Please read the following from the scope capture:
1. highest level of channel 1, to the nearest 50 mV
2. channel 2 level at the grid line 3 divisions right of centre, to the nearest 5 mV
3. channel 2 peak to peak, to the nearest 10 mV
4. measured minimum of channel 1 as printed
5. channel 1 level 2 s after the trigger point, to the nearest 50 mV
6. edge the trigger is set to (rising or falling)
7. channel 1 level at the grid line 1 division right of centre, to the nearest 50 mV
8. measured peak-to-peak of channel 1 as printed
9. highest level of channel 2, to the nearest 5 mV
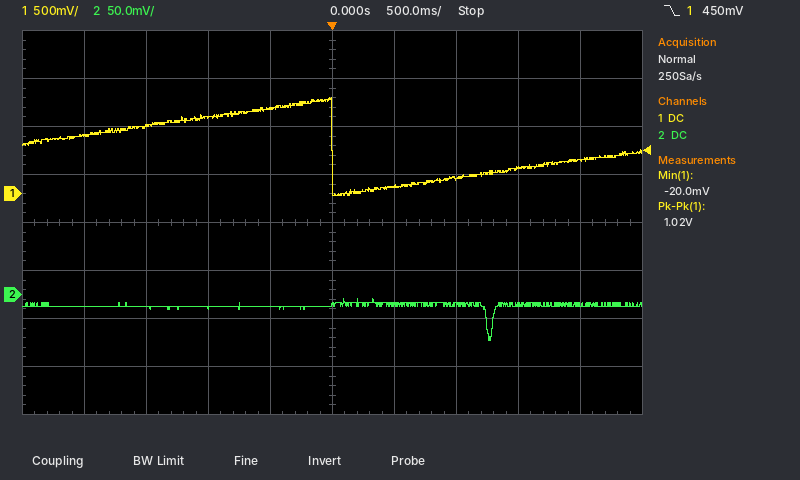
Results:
1.00 V
-10 mV
40 mV
-20.0 mV
350 mV
falling
100 mV
1.02 V
-5 mV
